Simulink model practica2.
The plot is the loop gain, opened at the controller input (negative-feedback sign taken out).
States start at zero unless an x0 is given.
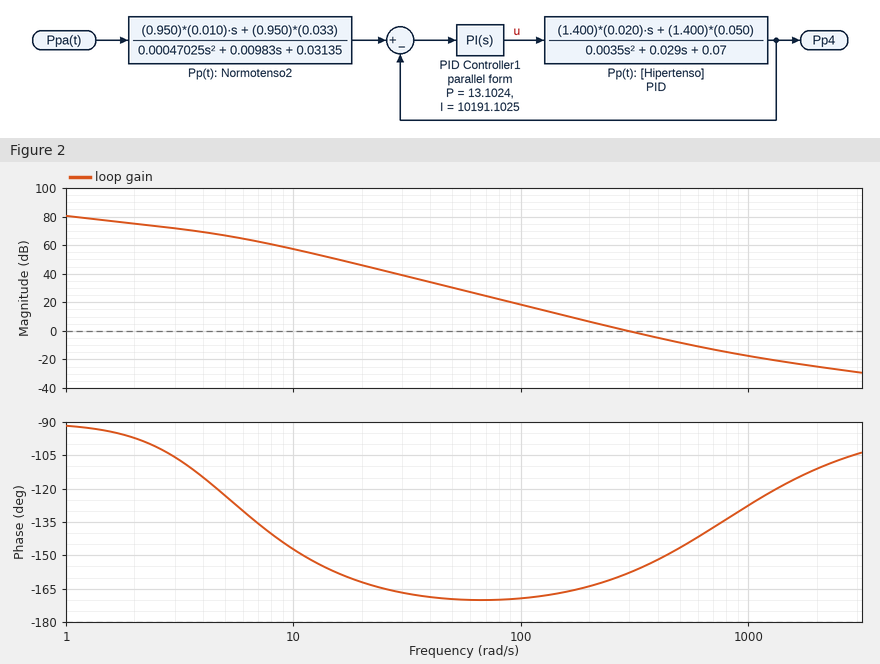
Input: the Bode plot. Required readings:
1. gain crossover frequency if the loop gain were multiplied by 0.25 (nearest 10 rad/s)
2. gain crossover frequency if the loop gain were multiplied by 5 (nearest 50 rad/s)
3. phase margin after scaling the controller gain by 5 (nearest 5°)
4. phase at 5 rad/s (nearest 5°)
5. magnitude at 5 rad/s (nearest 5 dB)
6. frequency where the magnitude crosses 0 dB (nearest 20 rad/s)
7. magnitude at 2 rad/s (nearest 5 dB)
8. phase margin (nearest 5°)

140 rad/s
750 rad/s
45°
-125°
65 dB
300 rad/s
75 dB
20°
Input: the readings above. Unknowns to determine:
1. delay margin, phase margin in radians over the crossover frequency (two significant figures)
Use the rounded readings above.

0.0012 s
